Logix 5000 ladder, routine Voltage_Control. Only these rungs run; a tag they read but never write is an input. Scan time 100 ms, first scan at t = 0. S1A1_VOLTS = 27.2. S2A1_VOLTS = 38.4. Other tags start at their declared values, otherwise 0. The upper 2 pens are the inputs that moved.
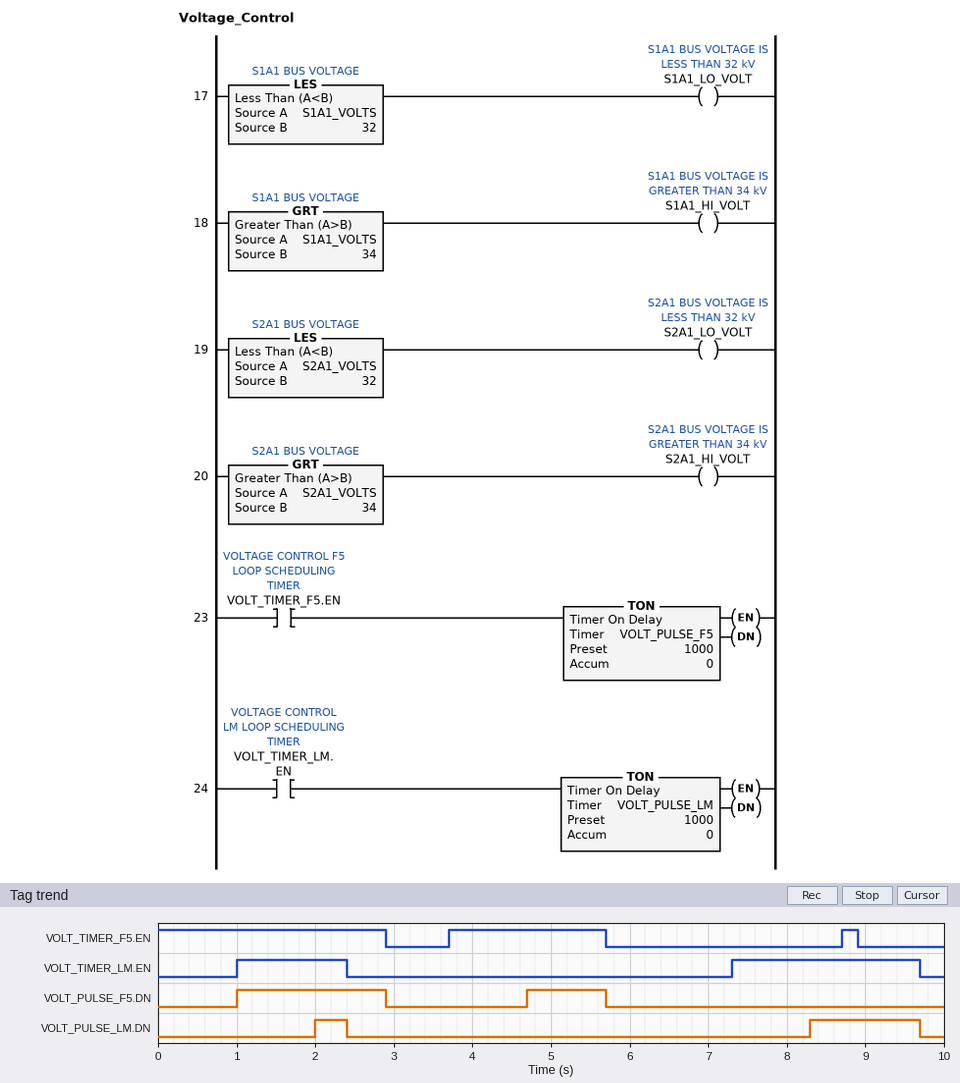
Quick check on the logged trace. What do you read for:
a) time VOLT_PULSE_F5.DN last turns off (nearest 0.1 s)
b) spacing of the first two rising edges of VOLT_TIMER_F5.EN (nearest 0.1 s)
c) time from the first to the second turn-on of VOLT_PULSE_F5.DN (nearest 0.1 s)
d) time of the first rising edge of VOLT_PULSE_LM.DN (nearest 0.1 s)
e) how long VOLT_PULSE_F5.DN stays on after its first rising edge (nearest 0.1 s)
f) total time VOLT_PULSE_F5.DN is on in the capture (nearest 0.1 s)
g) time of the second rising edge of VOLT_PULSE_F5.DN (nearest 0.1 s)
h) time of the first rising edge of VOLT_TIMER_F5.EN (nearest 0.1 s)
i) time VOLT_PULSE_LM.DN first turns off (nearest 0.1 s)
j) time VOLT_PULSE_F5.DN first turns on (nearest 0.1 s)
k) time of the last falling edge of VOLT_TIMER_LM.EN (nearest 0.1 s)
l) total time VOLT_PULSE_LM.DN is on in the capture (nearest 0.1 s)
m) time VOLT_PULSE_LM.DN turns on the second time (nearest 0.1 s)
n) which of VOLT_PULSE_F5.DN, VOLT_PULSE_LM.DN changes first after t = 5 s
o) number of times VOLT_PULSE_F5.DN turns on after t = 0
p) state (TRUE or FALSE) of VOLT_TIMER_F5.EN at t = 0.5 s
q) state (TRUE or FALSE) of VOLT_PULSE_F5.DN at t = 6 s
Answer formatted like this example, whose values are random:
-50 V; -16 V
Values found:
5.7 s; 5.0 s; 3.7 s; 2.0 s; 1.9 s; 2.9 s; 4.7 s; 3.7 s; 2.4 s; 1.0 s; 9.7 s; 1.8 s; 8.3 s; VOLT_PULSE_F5.DN; 2; TRUE; FALSE
